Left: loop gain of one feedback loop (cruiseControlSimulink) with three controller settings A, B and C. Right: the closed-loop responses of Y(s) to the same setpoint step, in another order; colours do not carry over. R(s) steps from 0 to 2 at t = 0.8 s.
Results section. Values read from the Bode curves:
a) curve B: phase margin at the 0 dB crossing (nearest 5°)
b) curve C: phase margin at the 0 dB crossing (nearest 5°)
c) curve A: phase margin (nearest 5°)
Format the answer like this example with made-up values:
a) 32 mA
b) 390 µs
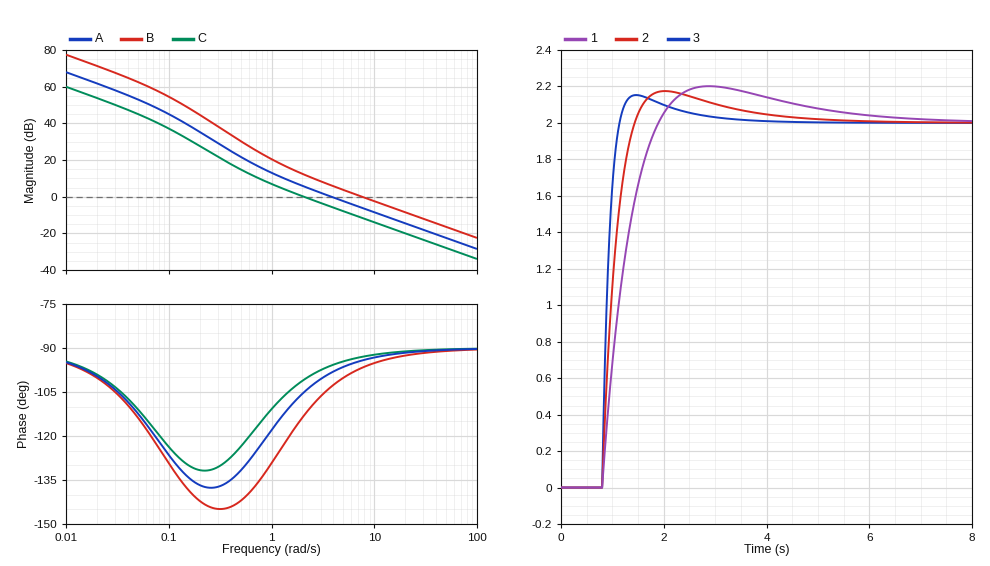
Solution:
a) 85°
b) 80°
c) 80°
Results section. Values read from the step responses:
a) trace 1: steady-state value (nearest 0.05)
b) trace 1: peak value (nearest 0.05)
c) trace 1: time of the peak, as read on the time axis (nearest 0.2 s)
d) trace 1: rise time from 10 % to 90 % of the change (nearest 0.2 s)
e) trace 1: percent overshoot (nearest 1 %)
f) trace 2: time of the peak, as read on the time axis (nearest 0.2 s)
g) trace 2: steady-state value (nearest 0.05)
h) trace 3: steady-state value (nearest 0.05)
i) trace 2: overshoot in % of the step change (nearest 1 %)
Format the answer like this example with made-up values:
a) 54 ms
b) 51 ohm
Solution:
a) 2.00
b) 2.20
c) 2.8 s
d) 0.8 s
e) 10 %
f) 2.0 s
g) 2.00
h) 2.00
i) 9 %
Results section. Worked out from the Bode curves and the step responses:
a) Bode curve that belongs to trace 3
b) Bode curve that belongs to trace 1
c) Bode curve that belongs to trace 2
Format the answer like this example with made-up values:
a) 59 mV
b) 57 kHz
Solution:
a) B
b) C
c) A
